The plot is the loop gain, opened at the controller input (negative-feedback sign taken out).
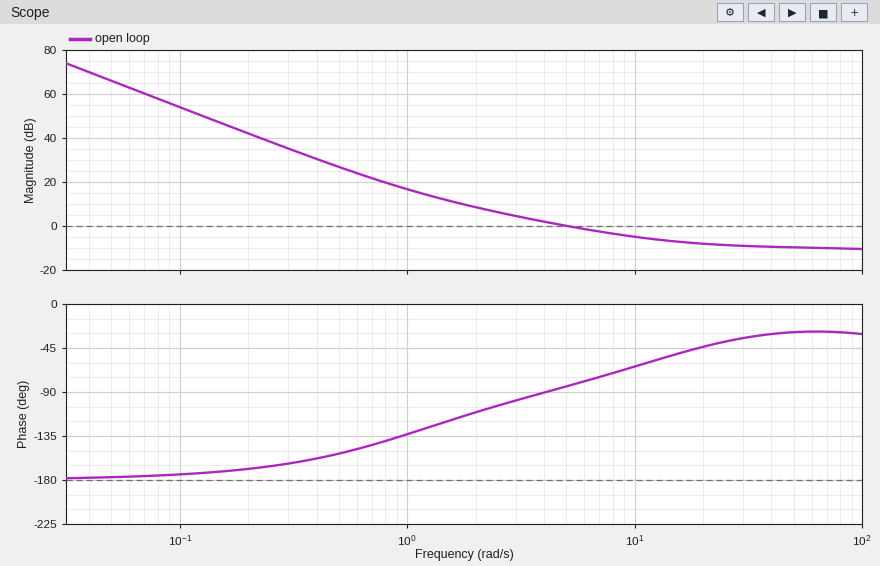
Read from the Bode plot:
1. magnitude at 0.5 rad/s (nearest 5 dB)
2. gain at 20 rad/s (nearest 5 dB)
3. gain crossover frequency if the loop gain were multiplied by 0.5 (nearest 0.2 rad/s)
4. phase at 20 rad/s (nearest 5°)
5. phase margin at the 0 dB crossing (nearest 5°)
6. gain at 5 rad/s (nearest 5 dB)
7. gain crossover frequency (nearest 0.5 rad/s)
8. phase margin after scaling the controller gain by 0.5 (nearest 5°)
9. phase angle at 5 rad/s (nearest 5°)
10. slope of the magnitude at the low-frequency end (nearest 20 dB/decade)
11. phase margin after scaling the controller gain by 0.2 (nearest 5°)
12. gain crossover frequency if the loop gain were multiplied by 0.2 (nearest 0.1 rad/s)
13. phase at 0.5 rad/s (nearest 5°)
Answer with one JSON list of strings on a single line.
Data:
["25 dB", "-10 dB", "2.6 rad/s", "-45°", "95°", "0 dB", "5.0 rad/s", "75°", "-85°", "-40 dB/decade", "55°", "1.2 rad/s", "-155°"]
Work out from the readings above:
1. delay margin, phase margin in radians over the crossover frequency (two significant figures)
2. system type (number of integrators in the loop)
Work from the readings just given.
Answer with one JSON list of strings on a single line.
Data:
["0.33 s", "2"]
